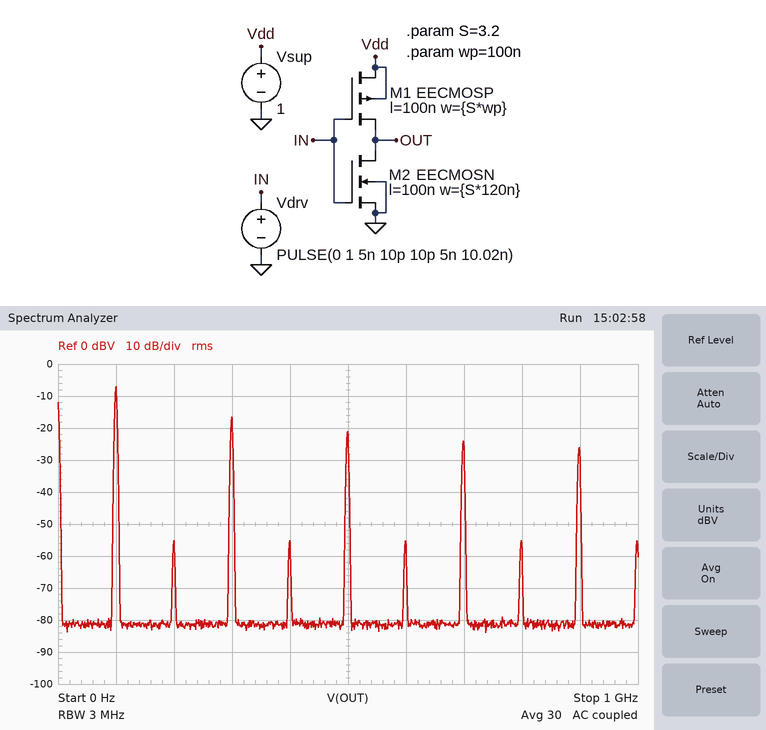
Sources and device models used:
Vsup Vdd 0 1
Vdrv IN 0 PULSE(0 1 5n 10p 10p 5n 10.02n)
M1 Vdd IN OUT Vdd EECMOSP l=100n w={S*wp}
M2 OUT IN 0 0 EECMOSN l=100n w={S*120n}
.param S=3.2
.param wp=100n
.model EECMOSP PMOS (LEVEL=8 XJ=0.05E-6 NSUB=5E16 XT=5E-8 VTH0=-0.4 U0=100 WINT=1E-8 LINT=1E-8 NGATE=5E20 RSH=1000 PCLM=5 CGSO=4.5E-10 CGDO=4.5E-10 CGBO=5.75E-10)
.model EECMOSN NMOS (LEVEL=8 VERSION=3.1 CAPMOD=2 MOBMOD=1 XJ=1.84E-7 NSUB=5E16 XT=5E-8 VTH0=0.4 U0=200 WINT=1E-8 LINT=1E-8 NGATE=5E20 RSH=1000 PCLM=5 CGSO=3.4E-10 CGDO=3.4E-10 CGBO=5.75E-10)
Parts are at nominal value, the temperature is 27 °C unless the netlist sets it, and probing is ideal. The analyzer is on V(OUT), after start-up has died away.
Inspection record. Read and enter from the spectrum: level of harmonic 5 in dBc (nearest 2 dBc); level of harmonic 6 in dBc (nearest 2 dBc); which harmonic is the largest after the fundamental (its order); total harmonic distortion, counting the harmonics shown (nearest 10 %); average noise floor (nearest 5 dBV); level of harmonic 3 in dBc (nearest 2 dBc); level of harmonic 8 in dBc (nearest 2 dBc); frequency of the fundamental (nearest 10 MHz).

-14 dBc
-48 dBc
3
40 %
-80 dBV
-10 dBc
-48 dBc
100 MHz
